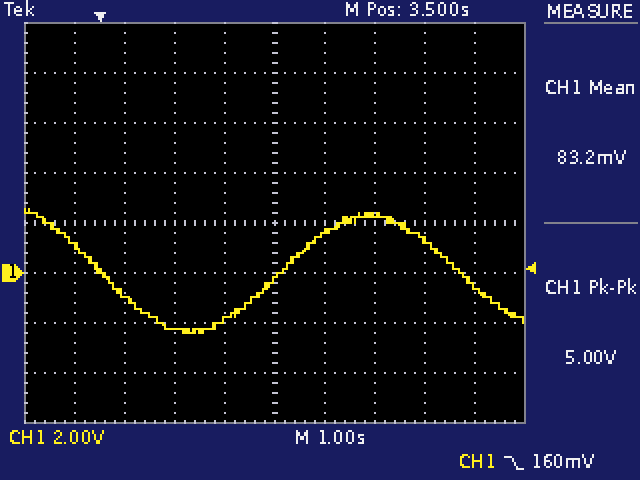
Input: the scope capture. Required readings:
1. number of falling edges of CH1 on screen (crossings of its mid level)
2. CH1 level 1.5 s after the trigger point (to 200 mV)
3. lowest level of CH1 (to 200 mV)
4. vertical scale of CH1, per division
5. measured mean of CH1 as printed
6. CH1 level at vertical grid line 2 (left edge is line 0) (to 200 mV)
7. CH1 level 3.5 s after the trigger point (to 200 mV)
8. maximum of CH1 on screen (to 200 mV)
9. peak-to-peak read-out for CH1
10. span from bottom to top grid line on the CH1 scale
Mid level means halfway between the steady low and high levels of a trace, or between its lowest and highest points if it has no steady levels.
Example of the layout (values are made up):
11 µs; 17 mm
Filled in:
2; -2.2 V; -2.4 V; 2 V; 83.2 mV; -800 mV; -200 mV; 2.6 V; 5.00 V; 16 V
